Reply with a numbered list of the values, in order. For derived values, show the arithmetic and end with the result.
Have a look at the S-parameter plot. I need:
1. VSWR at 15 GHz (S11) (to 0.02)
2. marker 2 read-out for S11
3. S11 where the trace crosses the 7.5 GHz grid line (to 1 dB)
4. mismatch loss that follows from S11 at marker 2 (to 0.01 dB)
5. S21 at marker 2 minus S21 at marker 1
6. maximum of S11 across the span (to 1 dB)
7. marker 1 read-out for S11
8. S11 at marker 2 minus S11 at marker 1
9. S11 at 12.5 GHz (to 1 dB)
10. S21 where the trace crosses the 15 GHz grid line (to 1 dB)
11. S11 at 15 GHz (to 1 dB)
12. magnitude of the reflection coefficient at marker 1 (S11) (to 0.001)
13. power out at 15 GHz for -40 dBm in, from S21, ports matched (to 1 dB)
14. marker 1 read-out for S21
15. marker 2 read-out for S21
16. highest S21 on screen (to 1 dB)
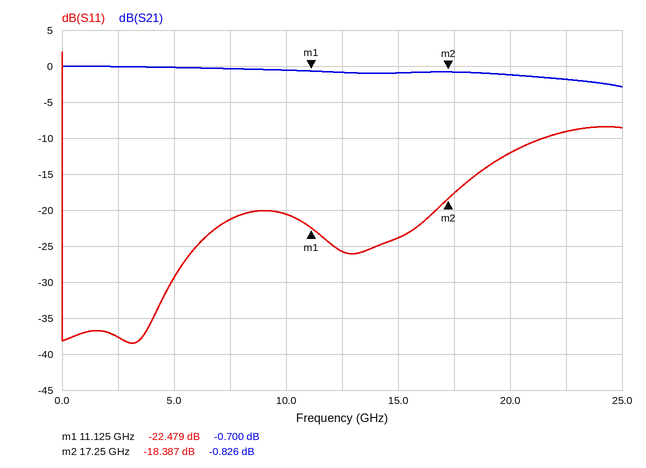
1. |Γ| = 10^(-24/20) = 0.0631; VSWR = (1 + 0.0631)/(1 − 0.0631) ≈ 1.13, so 1.14 to the nearest 0.02
2. -18.387 dB
3. -21 dB
4. −10 log10(1 − 10^(-18.387/10)) ≈ 0.06 dB
5. -0.826 − (-0.7) = -0.126 dB
6. 2 dB
7. -22.479 dB
8. -18.387 − (-22.479) = 4.092 dB
9. -26 dB
10. -1 dB
11. -24 dB
12. 10^(-22.479/20) ≈ 0.075
13. -40 dBm + (-1 dB) = -41 dBm
14. -0.700 dB
15. -0.826 dB
16. 0 dB
